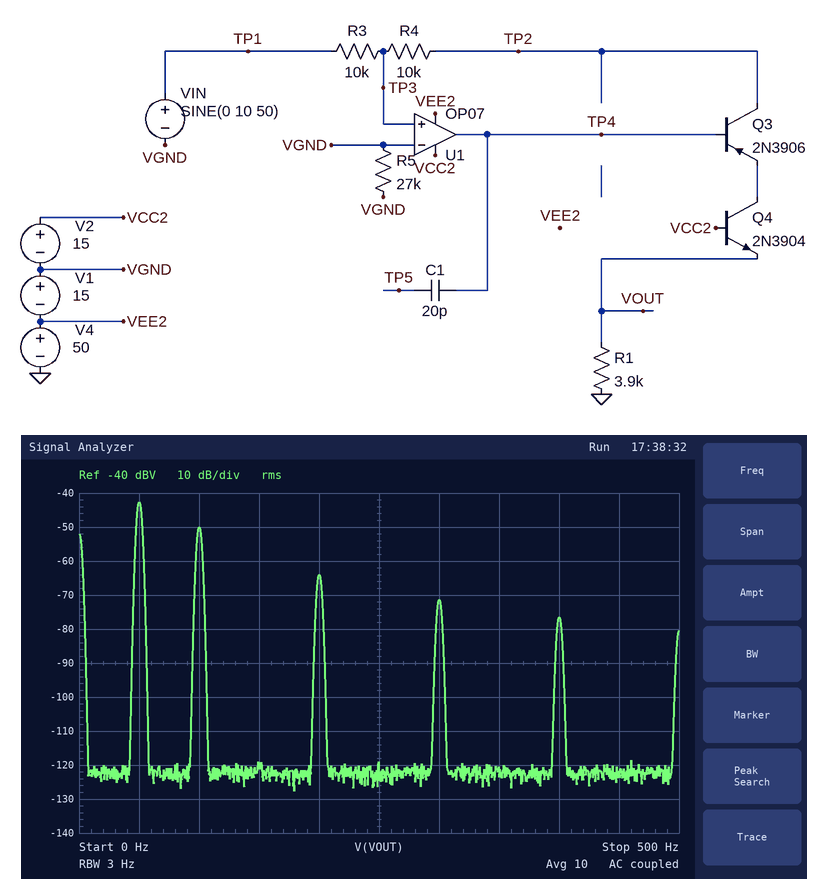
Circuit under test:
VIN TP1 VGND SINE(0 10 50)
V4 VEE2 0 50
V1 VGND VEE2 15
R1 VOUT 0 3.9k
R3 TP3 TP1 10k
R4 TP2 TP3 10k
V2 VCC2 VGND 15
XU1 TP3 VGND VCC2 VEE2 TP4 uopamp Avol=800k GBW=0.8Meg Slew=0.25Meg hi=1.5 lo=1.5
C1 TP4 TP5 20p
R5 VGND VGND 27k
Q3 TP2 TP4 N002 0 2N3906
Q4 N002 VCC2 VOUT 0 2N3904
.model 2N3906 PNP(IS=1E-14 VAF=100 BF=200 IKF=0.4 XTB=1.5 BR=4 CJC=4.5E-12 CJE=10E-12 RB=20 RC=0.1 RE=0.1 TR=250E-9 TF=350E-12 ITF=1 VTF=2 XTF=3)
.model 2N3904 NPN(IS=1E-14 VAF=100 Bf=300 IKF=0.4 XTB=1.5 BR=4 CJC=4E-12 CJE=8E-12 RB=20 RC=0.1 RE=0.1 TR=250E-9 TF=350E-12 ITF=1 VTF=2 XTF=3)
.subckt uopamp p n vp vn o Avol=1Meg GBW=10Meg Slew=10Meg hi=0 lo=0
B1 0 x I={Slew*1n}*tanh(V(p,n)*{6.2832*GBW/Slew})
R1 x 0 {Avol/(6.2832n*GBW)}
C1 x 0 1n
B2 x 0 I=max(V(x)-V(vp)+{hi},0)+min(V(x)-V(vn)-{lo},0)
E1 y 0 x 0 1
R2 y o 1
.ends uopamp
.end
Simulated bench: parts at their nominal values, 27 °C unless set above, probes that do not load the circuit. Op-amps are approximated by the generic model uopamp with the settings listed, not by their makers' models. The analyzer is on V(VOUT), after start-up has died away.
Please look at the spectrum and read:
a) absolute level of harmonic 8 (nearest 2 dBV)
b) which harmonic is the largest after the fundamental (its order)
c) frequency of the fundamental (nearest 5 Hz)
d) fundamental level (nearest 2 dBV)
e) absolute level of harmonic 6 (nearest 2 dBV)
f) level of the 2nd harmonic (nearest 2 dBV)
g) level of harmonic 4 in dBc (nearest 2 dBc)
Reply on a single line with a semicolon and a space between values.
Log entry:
-76 dBV; 2; 50 Hz; -42 dBV; -72 dBV; -50 dBV; -22 dBc
